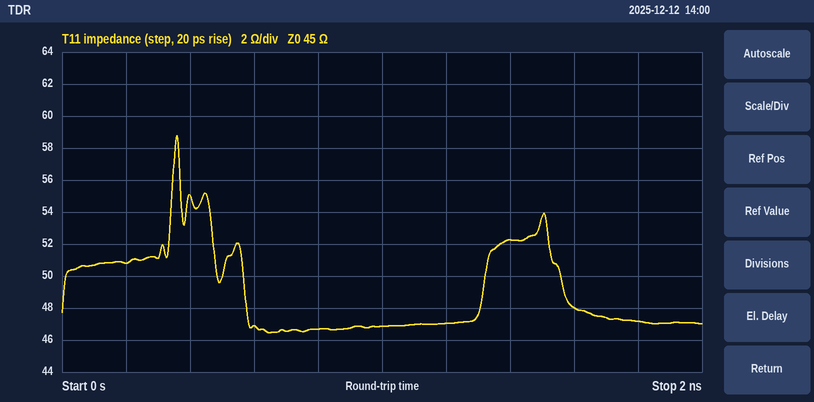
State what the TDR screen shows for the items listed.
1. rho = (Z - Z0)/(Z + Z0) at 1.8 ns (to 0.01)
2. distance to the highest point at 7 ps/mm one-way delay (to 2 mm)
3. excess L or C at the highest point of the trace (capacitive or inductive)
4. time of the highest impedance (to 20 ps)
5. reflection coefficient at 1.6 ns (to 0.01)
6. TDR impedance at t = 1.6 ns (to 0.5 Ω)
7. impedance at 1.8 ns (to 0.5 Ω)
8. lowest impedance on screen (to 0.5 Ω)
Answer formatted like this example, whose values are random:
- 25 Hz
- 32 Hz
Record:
- +0.02
- 26 mm
- inductive
- 360 ps
- +0.03
- 48.0 Ω
- 47.0 Ω
- 46.5 Ω
